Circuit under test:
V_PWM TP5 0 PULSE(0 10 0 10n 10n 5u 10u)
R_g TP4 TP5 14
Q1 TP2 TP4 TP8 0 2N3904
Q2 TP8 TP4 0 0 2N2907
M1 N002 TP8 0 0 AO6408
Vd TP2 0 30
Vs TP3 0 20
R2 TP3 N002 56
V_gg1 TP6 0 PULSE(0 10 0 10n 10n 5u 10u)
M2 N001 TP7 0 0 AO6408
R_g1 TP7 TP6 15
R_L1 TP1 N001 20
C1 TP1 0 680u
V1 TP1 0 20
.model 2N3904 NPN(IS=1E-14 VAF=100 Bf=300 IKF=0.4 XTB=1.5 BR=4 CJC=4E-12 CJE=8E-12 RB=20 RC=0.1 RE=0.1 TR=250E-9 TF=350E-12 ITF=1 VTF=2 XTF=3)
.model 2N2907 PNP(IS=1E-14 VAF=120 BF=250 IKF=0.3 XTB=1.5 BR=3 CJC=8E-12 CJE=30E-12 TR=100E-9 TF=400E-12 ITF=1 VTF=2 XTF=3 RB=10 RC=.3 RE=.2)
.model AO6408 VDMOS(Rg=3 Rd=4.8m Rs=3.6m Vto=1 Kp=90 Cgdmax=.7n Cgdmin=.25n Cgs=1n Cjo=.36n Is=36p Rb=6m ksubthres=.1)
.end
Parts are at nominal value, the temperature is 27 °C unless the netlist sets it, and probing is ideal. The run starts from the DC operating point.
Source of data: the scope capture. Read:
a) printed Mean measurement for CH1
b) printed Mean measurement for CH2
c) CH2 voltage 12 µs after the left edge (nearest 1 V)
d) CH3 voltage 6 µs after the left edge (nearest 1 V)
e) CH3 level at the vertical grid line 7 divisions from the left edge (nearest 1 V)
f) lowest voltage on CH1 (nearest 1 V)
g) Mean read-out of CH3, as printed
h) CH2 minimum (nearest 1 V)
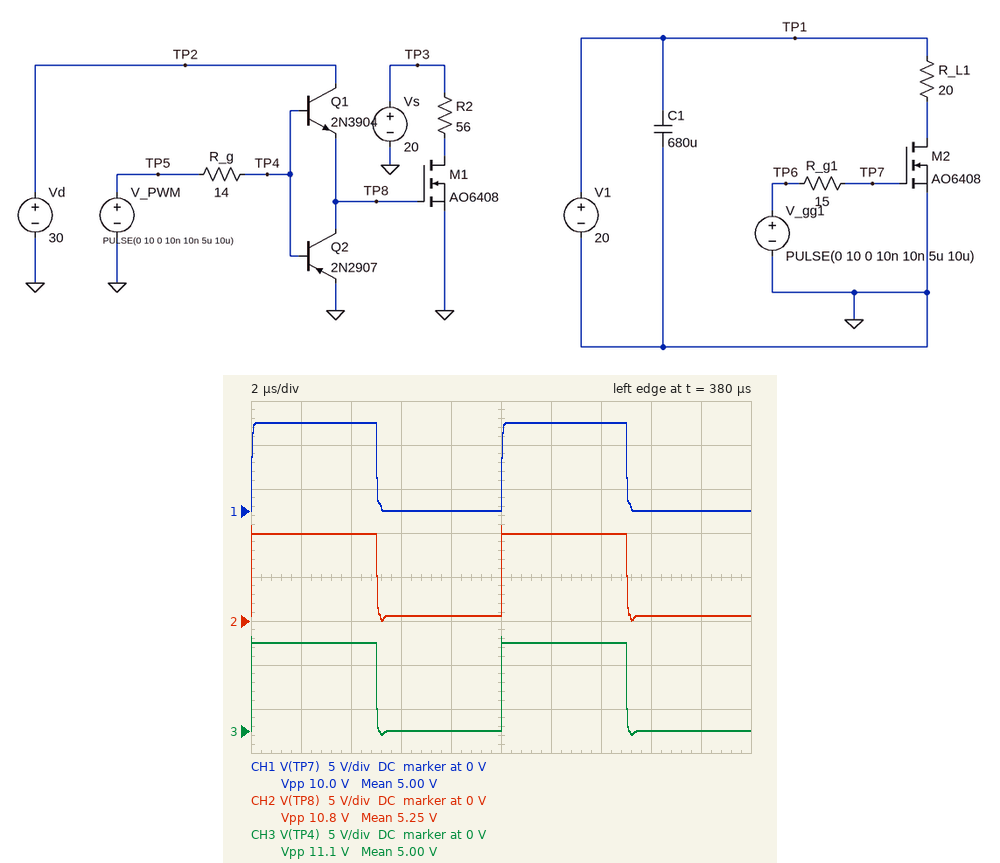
5.00 V
5.25 V
10 V
0 V
10 V
0 V
5.00 V
0 V
